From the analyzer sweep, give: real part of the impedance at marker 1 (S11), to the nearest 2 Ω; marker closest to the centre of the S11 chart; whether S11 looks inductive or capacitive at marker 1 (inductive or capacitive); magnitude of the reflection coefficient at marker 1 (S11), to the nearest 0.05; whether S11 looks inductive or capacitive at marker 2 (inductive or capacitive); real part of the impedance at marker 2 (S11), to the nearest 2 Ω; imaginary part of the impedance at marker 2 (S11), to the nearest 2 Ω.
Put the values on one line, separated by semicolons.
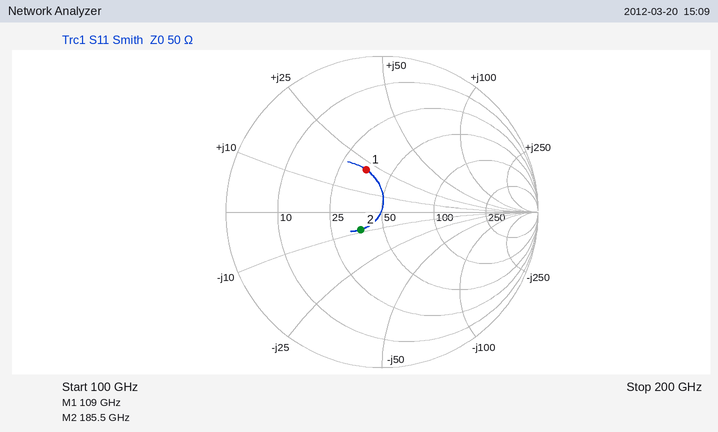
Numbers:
36 Ω; marker 2; inductive; 0.30; capacitive; 38 Ω; -8 Ω
